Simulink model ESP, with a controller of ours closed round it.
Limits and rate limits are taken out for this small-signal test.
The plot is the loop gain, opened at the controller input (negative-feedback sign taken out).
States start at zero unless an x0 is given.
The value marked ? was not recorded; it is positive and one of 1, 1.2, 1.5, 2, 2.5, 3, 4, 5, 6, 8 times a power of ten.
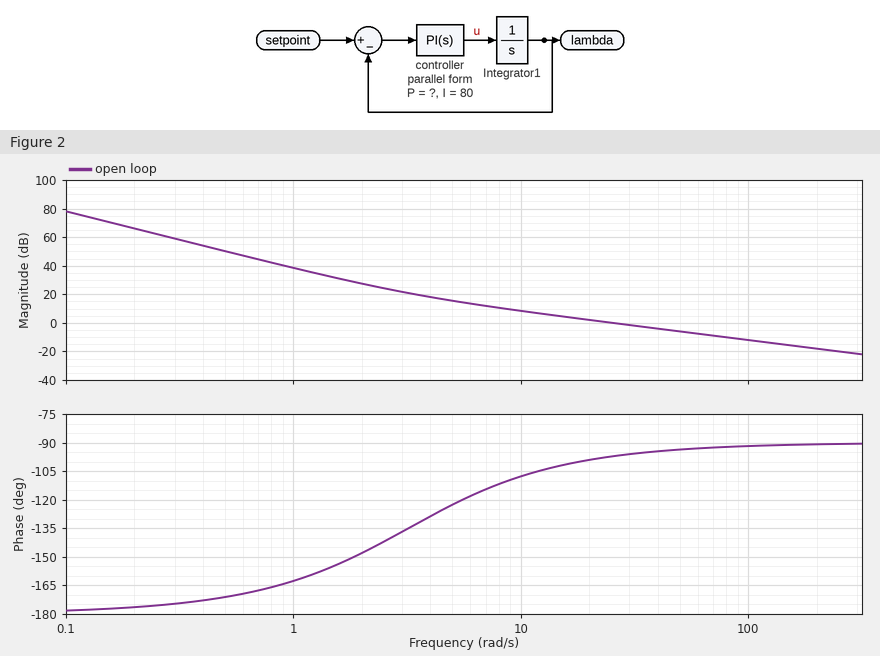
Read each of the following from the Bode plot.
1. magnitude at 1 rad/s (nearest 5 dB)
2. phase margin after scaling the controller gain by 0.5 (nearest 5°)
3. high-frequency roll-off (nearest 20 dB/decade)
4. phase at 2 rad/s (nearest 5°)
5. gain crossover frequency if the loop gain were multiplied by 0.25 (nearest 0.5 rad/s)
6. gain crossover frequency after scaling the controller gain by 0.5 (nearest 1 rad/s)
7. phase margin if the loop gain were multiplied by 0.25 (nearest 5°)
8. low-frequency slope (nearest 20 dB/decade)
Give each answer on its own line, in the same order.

40 dB
75°
-20 dB/decade
-150°
7.0 rad/s
13 rad/s
65°
-40 dB/decade
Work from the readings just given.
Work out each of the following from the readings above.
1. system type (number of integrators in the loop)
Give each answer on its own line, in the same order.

2
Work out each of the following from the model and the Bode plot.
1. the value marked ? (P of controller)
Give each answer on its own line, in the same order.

25
